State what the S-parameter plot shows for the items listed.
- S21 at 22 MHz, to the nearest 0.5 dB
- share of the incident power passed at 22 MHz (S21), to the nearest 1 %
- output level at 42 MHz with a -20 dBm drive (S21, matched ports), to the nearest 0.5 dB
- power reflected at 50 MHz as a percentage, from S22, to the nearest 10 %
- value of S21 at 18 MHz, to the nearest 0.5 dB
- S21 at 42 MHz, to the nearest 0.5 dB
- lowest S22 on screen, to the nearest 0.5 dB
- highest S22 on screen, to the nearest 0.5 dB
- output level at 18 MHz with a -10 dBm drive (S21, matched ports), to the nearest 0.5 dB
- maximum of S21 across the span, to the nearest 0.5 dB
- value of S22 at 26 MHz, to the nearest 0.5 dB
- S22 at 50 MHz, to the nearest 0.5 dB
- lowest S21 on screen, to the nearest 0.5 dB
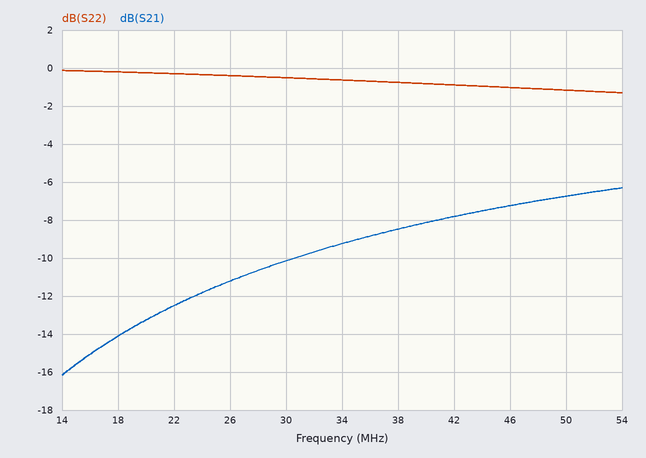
-12.5 dB
6 %
-28.0 dBm
80 %
-14.0 dB
-8.0 dB
-1.5 dB
0.0 dB
-24.0 dBm
-6.5 dB
-0.5 dB
-1.0 dB
-16.0 dB
